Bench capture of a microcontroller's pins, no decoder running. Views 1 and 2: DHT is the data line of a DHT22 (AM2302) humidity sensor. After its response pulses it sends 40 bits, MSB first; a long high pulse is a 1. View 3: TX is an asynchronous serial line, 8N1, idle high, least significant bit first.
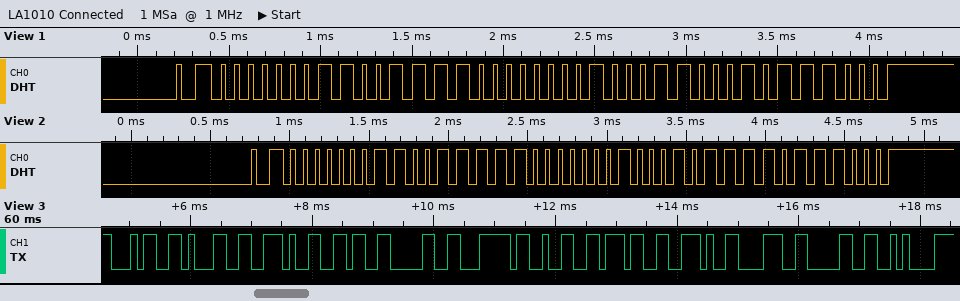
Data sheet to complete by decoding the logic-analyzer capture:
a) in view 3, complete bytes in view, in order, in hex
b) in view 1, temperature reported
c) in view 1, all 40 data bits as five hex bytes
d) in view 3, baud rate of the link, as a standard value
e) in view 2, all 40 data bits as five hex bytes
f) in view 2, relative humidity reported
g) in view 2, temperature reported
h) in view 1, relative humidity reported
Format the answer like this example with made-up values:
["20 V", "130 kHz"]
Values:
["34 31 2E 36 30 7C 32 37 2E 38 30 0A", "28.0 °C", "01 9E 01 18 B8", "9600 baud", "01 9F 01 17 B8", "41.5 %", "27.9 °C", "41.4 %"]
